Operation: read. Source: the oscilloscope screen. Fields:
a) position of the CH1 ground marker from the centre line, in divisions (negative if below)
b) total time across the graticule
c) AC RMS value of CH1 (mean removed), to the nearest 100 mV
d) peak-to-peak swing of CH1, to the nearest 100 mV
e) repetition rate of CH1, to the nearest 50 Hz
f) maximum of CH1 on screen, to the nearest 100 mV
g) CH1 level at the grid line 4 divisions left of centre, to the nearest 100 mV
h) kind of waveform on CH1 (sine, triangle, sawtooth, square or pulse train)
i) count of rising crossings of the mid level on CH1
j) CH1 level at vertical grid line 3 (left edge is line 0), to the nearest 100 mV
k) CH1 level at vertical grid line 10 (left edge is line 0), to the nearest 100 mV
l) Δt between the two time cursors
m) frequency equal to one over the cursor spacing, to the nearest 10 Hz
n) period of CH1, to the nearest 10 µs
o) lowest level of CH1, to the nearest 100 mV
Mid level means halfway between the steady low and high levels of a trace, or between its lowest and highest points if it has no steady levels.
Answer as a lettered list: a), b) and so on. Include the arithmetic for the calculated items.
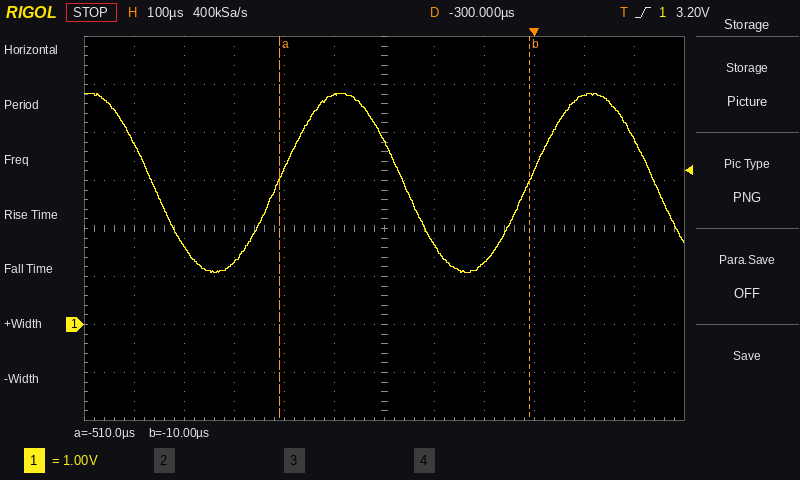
a) -2.0 div
b) 1.2 ms
c) 3.7 V / (2√2) ≈ 1.3 V
d) 4.8 V − (1.1 V) = 3.7 V
e) 1 / 500 µs ≈ 2.00 kHz
f) 4.8 V
g) 1.6 V
h) sine
i) 2
j) 1.3 V
k) 4.8 V
l) -10 µs − (-510 µs) = 500 µs
m) 1 / 500 µs ≈ 2.00 kHz
n) 500 µs
o) 1.1 V
